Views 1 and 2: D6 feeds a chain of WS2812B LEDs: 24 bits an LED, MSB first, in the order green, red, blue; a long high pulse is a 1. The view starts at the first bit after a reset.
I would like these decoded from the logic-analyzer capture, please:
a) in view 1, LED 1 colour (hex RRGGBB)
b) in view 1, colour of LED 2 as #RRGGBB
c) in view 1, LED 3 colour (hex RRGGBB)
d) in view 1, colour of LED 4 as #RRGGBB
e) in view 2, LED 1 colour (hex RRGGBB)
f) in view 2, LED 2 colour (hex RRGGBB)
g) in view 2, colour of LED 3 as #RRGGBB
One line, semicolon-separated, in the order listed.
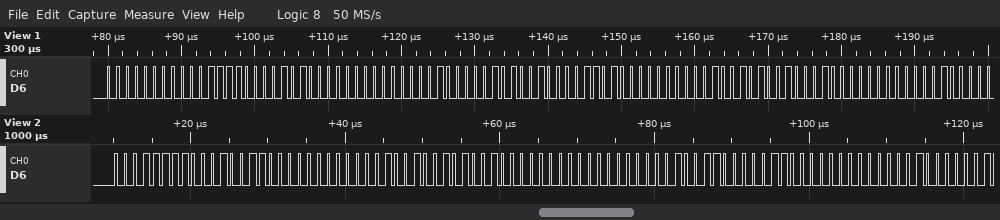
#1E0014; #080029; #000D25; #002210; #131F00; #290900; #26000C
